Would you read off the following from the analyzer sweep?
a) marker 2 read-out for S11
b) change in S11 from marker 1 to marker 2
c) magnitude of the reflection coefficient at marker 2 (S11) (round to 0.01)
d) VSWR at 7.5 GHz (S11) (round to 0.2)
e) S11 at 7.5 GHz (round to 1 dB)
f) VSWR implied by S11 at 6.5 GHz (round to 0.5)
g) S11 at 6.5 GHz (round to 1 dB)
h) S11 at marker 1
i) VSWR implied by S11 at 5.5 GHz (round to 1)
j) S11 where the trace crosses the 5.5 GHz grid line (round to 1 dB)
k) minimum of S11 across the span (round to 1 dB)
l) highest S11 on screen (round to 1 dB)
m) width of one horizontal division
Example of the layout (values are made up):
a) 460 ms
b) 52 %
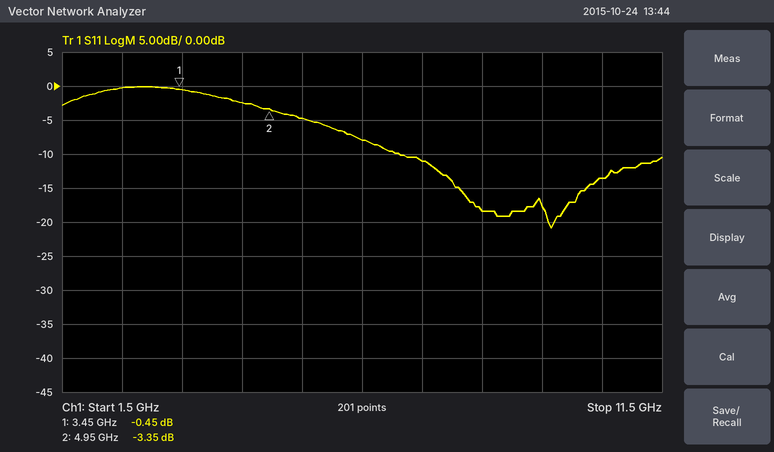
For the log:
a) -3.35 dB
b) -2.90 dB
c) 0.68
d) 1.8
e) -11 dB
f) 2.5
g) -8 dB
h) -0.45 dB
i) 4
j) -5 dB
k) -21 dB
l) 0 dB
m) 1 GHz
